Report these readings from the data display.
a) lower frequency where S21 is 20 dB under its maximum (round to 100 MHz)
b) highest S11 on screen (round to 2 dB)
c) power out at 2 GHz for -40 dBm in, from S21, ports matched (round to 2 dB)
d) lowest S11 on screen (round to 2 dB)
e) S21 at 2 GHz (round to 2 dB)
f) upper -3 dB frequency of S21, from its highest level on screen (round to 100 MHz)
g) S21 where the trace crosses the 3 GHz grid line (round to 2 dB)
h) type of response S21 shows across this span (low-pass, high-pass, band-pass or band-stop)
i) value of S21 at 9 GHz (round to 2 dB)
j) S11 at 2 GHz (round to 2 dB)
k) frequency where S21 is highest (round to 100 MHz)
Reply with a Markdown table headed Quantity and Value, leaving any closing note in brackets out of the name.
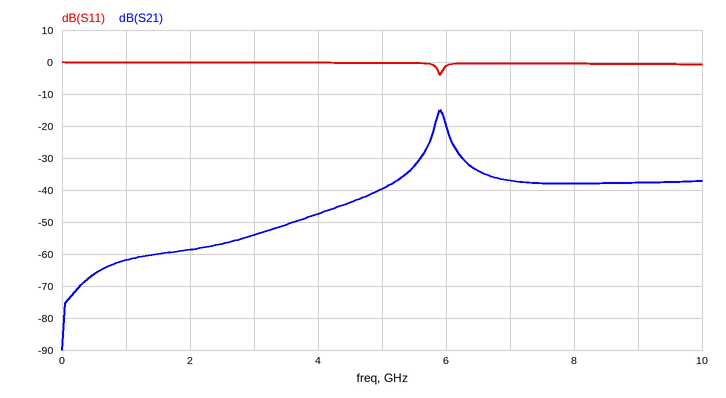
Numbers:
| Quantity | Value |
|---|---|
| lower frequency where S21 is 20 dB under its maximum | 5.4 GHz |
| highest S11 on screen | 0 dB |
| power out at 2 GHz for -40 dBm in, from S21, ports matched | -98 dBm |
| lowest S11 on screen | -4 dB |
| S21 at 2 GHz | -58 dB |
| upper -3 dB frequency of S21, from its highest level on screen | 6.0 GHz |
| S21 where the trace crosses the 3 GHz grid line | -54 dB |
| type of response S21 shows across this span | band-pass |
| value of S21 at 9 GHz | -38 dB |
| S11 at 2 GHz | 0 dB |
| frequency where S21 is highest | 5.9 GHz |
